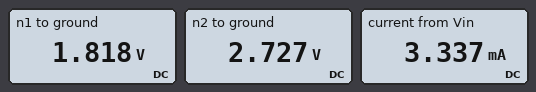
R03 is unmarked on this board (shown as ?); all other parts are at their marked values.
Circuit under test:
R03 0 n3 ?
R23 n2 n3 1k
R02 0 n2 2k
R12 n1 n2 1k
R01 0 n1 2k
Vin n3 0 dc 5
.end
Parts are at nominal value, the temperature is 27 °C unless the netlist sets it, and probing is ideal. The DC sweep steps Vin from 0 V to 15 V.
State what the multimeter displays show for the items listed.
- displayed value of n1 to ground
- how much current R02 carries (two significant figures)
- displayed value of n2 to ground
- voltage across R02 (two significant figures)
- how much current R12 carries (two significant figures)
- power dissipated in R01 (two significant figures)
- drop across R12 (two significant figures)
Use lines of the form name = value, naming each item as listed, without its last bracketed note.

displayed value of n1 to ground = 1.818 V
how much current R02 carries = 1.4 mA
displayed value of n2 to ground = 2.727 V
voltage across R02 = 2.7 V
how much current R12 carries = 910 µA
power dissipated in R01 = 1.7 mW
drop across R12 = 910 mV
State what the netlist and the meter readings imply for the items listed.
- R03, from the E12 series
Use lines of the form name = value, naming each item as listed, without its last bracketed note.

R03, from the E12 series = 4.7 kΩ
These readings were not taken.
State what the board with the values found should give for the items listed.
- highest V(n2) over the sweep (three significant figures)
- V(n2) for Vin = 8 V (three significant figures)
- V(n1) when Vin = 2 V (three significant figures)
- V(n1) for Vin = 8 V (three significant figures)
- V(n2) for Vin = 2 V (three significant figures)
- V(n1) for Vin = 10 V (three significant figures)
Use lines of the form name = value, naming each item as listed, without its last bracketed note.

highest V(n2) over the sweep = 8.18 V
V(n2) for Vin = 8 V = 4.36 V
V(n1) when Vin = 2 V = 727 mV
V(n1) for Vin = 8 V = 2.91 V
V(n2) for Vin = 2 V = 1.09 V
V(n1) for Vin = 10 V = 3.64 V
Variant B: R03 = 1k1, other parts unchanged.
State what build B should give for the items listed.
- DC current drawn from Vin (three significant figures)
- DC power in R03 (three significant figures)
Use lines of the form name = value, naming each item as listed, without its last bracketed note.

DC current drawn from Vin = 6.82 mA
DC power in R03 = 22.7 mW
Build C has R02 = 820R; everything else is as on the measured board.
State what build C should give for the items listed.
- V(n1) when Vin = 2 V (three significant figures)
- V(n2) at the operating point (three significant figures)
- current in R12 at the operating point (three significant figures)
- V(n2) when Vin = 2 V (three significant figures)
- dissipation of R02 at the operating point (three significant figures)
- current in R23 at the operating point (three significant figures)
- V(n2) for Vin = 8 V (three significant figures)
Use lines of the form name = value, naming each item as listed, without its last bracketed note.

V(n1) when Vin = 2 V = 522 mV
V(n2) at the operating point = 1.96 V
current in R12 at the operating point = 653 µA
V(n2) when Vin = 2 V = 783 mV
dissipation of R02 at the operating point = 4.68 mW
current in R23 at the operating point = 3.04 mA
V(n2) for Vin = 8 V = 3.13 V
